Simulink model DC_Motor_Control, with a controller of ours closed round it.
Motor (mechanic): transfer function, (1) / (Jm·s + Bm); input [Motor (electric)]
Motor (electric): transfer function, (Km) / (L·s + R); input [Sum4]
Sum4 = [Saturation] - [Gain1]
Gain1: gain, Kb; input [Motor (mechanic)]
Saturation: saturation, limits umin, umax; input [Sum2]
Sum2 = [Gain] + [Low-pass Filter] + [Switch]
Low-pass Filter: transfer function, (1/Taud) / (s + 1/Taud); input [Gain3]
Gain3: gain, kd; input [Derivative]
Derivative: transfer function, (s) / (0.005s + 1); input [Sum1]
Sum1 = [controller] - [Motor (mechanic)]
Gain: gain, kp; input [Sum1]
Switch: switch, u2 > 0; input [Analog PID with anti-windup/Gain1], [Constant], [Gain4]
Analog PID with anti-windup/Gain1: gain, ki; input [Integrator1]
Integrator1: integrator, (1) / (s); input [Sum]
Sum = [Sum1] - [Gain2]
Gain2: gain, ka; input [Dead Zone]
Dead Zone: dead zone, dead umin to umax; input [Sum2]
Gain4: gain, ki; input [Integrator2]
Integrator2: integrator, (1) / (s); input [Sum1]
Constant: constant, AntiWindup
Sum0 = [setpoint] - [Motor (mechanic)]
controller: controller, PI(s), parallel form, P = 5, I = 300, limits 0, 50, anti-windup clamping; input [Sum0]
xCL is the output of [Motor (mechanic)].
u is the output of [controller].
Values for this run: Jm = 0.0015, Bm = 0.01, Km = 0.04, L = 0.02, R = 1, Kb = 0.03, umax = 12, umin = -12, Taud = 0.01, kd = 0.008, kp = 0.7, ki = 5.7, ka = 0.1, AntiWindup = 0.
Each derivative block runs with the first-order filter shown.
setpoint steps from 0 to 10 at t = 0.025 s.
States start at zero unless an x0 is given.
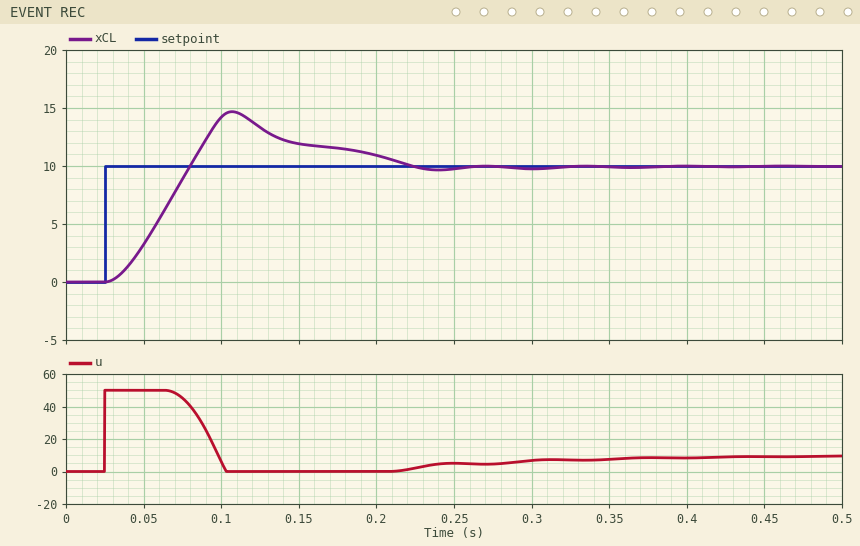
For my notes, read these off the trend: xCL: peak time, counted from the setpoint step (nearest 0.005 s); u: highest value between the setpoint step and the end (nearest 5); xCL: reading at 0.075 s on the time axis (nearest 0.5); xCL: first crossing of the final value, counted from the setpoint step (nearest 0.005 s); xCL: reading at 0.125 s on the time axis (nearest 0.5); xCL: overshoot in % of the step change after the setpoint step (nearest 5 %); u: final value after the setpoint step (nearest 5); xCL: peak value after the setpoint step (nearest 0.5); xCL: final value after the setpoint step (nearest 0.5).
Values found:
0.080 s
50
9.0
0.055 s
13.5
45 %
10
14.5
10.0
